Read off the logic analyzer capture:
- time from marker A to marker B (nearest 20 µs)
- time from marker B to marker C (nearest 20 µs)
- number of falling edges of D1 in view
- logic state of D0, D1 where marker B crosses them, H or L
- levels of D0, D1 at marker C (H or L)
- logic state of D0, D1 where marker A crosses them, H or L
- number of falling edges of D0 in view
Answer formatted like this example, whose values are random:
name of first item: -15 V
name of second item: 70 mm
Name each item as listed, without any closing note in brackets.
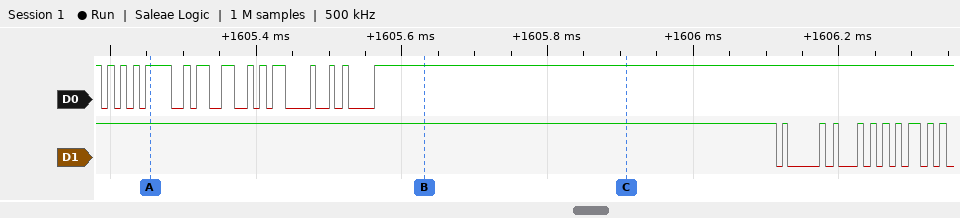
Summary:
time from marker A to marker B: 380 µs
time from marker B to marker C: 280 µs
number of falling edges of D1 in view: 11
logic state of D0, D1 where marker B crosses them, H or L: D0=H, D1=H
levels of D0, D1 at marker C: D0=H, D1=H
logic state of D0, D1 where marker A crosses them, H or L: D0=H, D1=H
number of falling edges of D0 in view: 14
